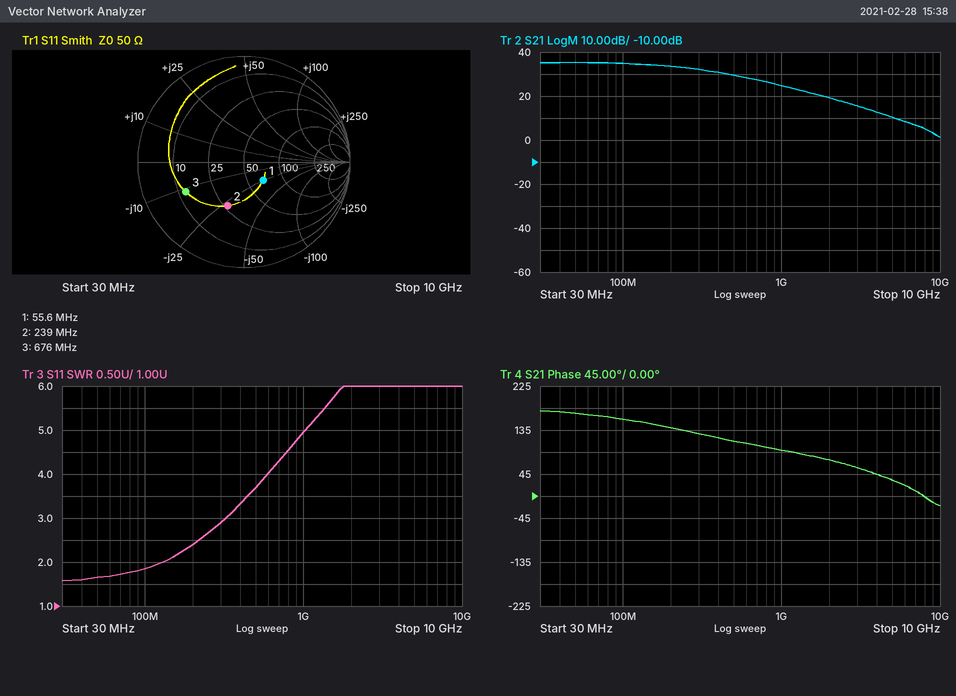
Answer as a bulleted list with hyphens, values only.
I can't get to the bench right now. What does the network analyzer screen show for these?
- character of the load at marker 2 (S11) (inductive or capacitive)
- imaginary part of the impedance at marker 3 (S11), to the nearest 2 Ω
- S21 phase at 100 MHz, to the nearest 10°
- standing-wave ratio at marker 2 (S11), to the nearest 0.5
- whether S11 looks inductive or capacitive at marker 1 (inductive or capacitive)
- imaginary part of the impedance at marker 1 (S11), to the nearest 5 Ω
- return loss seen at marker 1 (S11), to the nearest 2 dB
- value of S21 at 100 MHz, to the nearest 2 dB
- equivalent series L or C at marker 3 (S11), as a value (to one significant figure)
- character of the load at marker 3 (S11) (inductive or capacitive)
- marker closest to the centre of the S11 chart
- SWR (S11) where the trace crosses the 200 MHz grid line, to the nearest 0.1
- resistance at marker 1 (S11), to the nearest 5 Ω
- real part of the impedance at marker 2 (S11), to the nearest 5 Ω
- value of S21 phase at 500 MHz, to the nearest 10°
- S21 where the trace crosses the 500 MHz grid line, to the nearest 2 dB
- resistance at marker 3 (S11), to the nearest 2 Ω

- capacitive
- -12 Ω
- 160°
- 2.5
- capacitive
- -25 Ω
- 12 dB
- 34 dB
- 20 pF
- capacitive
- marker 1
- 2.4
- 65 Ω
- 25 Ω
- 110°
- 30 dB
- 12 Ω
